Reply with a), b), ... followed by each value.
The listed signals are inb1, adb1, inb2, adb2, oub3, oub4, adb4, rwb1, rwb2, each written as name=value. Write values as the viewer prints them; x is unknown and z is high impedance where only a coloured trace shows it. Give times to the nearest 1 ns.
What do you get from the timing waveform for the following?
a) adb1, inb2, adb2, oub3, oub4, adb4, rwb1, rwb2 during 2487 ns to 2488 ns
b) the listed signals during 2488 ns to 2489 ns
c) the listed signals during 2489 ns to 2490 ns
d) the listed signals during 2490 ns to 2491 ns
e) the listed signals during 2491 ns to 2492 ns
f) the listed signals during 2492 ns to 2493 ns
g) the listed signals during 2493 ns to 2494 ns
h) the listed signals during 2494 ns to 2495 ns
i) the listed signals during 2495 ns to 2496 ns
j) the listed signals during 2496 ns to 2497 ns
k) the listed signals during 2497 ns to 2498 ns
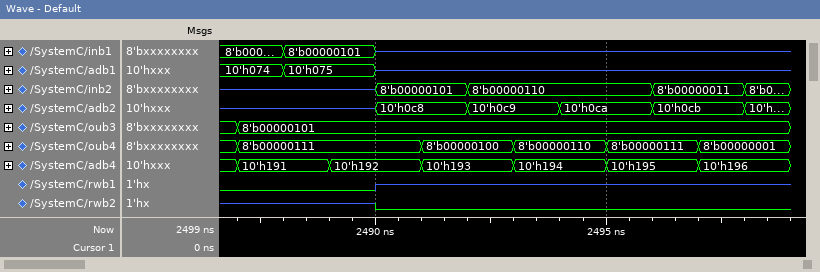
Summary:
a) adb1=10'h074, inb2=z, adb2=z, oub3=8'b00000101, oub4=8'b00000111, adb4=10'h191, rwb1=0, rwb2=z
b) inb1=8'b00000101, adb1=10'h075, inb2=z, adb2=z, oub3=8'b00000101, oub4=8'b00000111, adb4=10'h191, rwb1=0, rwb2=z
c) inb1=8'b00000101, adb1=10'h075, inb2=z, adb2=z, oub3=8'b00000101, oub4=8'b00000111, adb4=10'h192, rwb1=0, rwb2=z
d) inb1=z, adb1=z, inb2=8'b00000101, adb2=10'h0c8, oub3=8'b00000101, oub4=8'b00000111, adb4=10'h192, rwb1=z, rwb2=0
e) inb1=z, adb1=z, inb2=8'b00000101, adb2=10'h0c8, oub3=8'b00000101, oub4=8'b00000100, adb4=10'h193, rwb1=z, rwb2=0
f) inb1=z, adb1=z, inb2=8'b00000110, adb2=10'h0c9, oub3=8'b00000101, oub4=8'b00000100, adb4=10'h193, rwb1=z, rwb2=0
g) inb1=z, adb1=z, inb2=8'b00000110, adb2=10'h0c9, oub3=8'b00000101, oub4=8'b00000110, adb4=10'h194, rwb1=z, rwb2=0
h) inb1=z, adb1=z, inb2=8'b00000110, adb2=10'h0ca, oub3=8'b00000101, oub4=8'b00000110, adb4=10'h194, rwb1=z, rwb2=0
i) inb1=z, adb1=z, inb2=8'b00000110, adb2=10'h0ca, oub3=8'b00000101, oub4=8'b00000111, adb4=10'h195, rwb1=z, rwb2=0
j) inb1=z, adb1=z, inb2=8'b00000011, adb2=10'h0cb, oub3=8'b00000101, oub4=8'b00000111, adb4=10'h195, rwb1=z, rwb2=0
k) inb1=z, adb1=z, inb2=8'b00000011, adb2=10'h0cb, oub3=8'b00000101, oub4=8'b00000001, adb4=10'h196, rwb1=z, rwb2=0
